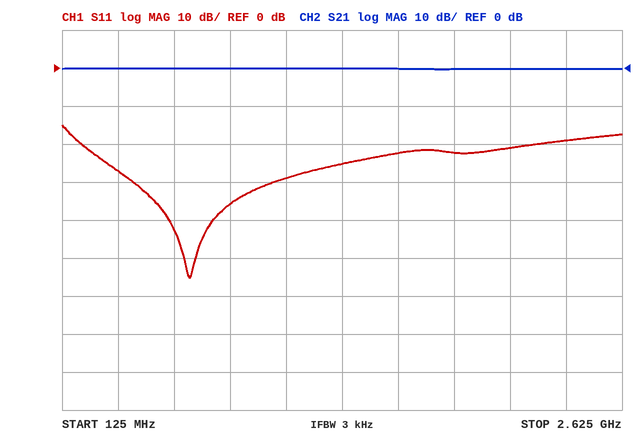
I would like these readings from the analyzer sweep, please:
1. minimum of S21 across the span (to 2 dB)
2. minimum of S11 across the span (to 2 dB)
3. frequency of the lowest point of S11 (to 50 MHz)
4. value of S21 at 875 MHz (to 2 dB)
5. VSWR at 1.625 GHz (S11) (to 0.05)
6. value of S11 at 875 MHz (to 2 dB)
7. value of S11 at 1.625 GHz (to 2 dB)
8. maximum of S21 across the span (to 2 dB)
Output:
0 dB
-56 dB
700 MHz
0 dB
1.15
-36 dB
-22 dB
0 dB
